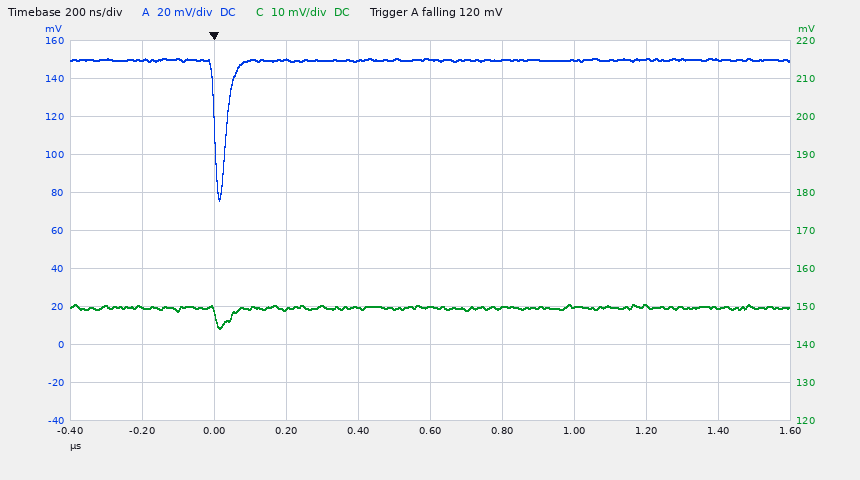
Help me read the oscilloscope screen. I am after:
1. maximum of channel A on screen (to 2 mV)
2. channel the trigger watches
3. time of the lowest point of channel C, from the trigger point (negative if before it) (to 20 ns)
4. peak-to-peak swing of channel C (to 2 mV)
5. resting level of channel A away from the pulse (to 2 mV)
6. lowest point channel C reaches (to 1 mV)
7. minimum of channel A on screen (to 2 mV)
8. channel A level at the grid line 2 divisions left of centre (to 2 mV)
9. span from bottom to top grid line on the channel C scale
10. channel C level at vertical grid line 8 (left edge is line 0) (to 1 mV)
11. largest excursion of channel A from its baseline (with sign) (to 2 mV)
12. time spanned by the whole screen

150 mV
channel A
+20 ns
6 mV
150 mV
144 mV
76 mV
150 mV
100 mV
150 mV
-74 mV
2 µs
